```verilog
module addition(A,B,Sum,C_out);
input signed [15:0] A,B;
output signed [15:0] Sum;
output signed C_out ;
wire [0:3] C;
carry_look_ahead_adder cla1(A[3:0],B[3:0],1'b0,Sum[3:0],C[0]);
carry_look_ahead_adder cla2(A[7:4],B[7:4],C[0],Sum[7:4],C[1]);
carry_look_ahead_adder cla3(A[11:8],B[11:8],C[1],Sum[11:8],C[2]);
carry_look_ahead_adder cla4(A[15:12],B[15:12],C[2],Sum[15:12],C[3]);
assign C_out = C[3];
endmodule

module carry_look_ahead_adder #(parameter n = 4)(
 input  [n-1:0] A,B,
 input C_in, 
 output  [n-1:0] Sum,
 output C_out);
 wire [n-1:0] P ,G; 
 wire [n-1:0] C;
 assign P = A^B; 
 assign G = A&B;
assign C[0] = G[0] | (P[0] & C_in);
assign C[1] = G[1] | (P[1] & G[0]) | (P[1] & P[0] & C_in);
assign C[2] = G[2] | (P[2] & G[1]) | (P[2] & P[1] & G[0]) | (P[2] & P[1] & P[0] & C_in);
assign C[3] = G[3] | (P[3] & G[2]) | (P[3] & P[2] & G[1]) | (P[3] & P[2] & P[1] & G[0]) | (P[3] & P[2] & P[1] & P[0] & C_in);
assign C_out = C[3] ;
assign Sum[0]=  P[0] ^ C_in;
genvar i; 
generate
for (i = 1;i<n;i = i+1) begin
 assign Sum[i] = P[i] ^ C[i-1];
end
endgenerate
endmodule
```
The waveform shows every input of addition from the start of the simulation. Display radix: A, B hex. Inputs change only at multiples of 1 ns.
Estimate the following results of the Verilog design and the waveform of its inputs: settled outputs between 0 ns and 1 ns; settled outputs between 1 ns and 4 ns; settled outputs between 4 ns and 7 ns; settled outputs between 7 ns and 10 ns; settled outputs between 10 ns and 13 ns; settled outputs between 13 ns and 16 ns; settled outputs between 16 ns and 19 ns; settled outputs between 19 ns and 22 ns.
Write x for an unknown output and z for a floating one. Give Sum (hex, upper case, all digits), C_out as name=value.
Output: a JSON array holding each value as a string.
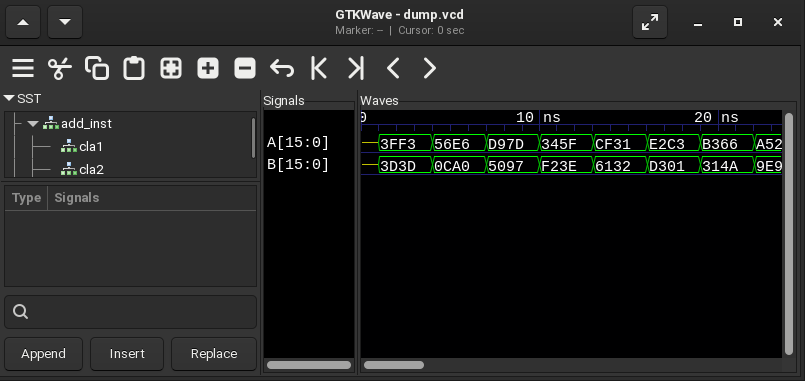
["Sum=x, C_out=x", "Sum=7D30, C_out=0", "Sum=6386, C_out=0", "Sum=2A14, C_out=1", "Sum=269D, C_out=1", "Sum=3063, C_out=1", "Sum=B5C4, C_out=1", "Sum=E4B0, C_out=0"]
